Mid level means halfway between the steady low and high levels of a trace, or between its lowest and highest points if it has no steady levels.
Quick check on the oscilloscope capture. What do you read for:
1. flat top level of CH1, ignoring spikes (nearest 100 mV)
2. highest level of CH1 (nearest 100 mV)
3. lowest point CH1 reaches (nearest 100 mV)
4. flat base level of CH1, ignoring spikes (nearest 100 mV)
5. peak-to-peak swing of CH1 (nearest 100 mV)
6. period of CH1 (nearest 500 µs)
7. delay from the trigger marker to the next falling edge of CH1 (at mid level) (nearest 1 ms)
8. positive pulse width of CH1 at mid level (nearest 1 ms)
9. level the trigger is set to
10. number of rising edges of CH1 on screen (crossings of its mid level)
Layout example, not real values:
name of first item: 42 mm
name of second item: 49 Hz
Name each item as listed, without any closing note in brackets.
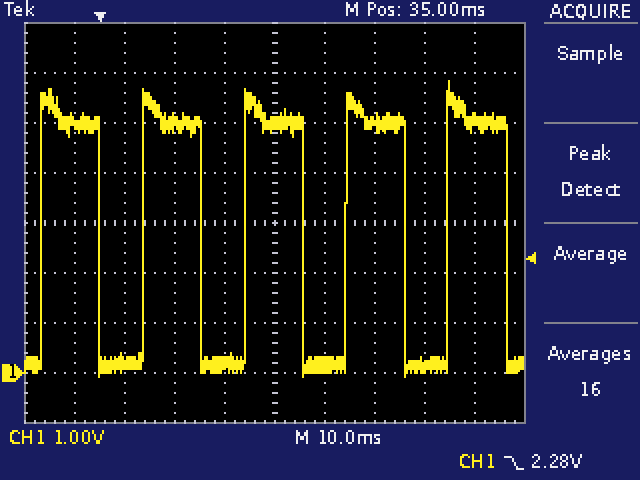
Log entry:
flat top level of CH1, ignoring spikes: 5.0 V
highest level of CH1: 5.8 V
lowest point CH1 reaches: -100 mV
flat base level of CH1, ignoring spikes: 200 mV
peak-to-peak swing of CH1: 5.9 V
period of CH1: 20.5 ms
delay from the trigger marker to the next falling edge of CH1 (at mid level): 20 ms
positive pulse width of CH1 at mid level: 12 ms
level the trigger is set to: 2.28 V
number of rising edges of CH1 on screen: 5
